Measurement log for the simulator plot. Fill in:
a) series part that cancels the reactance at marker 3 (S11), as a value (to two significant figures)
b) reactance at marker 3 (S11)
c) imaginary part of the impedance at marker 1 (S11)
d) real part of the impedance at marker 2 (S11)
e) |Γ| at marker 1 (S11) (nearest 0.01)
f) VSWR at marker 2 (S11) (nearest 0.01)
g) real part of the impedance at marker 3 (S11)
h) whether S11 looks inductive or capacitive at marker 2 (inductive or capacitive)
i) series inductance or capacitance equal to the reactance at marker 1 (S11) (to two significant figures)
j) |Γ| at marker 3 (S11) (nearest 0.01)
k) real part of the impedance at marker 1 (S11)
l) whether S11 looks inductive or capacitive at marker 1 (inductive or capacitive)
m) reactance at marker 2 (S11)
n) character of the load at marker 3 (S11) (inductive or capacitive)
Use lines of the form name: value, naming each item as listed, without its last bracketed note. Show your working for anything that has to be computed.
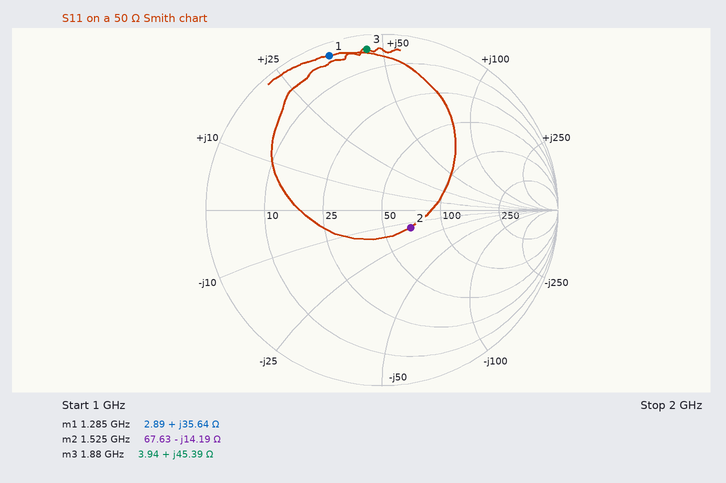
series part that cancels the reactance at marker 3 (S11), as a value: C = 1/(2π × 1.88 GHz × 45.39 Ω) ≈ 1.9 pF
reactance at marker 3: +45.39 Ω
imaginary part of the impedance at marker 1: +35.64 Ω
real part of the impedance at marker 2: 67.63 Ω
|Γ| at marker 1 (S11): 0.93
VSWR at marker 2 (S11): 1.47
real part of the impedance at marker 3: 3.94 Ω
whether S11 looks inductive or capacitive at marker 2: capacitive
series inductance or capacitance equal to the reactance at marker 1 (S11): L = 35.64 Ω/(2π × 1.285 GHz) ≈ 4.4 nH
|Γ| at marker 3 (S11): 0.92
real part of the impedance at marker 1: 2.89 Ω
whether S11 looks inductive or capacitive at marker 1: inductive
reactance at marker 2: -14.19 Ω
character of the load at marker 3 (S11): inductive
